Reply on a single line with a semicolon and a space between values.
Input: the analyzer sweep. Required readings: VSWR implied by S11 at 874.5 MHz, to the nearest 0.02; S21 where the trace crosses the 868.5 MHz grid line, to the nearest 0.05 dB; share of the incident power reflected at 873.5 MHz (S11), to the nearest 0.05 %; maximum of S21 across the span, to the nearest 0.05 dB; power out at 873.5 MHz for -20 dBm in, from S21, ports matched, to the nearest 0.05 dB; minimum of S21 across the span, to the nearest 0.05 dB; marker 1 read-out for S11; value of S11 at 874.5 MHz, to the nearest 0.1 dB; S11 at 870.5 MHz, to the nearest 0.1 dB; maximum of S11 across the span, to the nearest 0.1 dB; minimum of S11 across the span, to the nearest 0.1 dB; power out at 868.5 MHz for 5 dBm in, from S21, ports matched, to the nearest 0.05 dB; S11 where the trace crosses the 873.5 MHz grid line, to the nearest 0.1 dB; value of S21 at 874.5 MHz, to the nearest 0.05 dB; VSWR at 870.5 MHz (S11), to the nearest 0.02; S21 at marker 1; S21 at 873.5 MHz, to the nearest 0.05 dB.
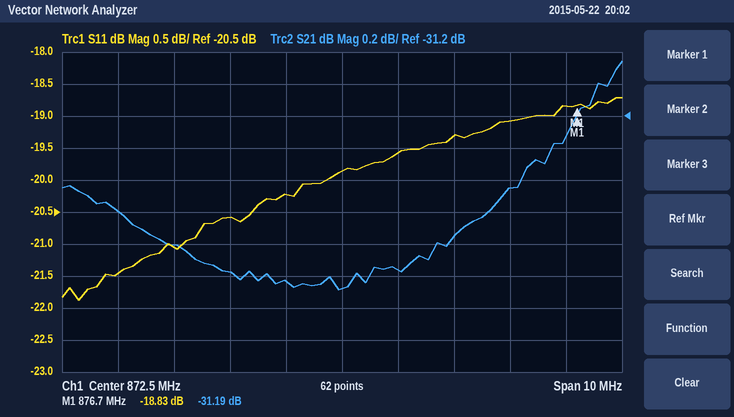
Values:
1.24; -31.80 dB; 1.10 %; -30.85 dB; -52.15 dBm; -32.30 dB; -18.83 dB; -19.3 dB; -20.6 dB; -18.7 dB; -21.9 dB; -26.80 dBm; -19.6 dB; -31.95 dB; 1.20; -31.19 dB; -32.15 dB
